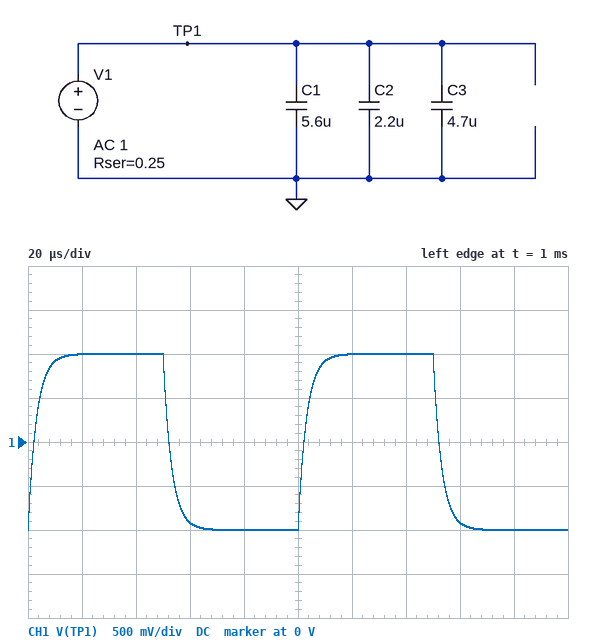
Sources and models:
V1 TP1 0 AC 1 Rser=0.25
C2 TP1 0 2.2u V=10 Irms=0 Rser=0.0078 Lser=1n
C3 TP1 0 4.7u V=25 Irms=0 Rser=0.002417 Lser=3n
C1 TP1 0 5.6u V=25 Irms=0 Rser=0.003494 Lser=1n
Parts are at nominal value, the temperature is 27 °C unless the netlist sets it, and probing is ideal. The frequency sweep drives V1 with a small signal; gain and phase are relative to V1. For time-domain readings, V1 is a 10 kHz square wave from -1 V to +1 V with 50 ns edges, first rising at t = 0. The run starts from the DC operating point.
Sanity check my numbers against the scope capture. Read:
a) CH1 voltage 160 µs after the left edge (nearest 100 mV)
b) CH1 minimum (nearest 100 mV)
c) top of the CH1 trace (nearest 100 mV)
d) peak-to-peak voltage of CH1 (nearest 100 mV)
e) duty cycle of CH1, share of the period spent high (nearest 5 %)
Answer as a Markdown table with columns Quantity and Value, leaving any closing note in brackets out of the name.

| Quantity | Value |
|---|---|
| CH1 voltage 160 µs after the left edge | -900 mV |
| CH1 minimum | -1.0 V |
| top of the CH1 trace | 1.0 V |
| peak-to-peak voltage of CH1 | 2.0 V |
| duty cycle of CH1, share of the period spent high | 50 % |
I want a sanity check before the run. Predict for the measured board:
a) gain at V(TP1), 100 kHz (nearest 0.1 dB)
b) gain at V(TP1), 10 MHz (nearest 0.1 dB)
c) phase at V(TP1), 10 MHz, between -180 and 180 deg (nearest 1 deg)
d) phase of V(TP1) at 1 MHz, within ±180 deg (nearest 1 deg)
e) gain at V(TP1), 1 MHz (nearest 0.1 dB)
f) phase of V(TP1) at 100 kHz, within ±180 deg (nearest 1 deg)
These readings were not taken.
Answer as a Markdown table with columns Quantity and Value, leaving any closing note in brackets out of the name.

| Quantity | Value |
|---|---|
| gain at V(TP1), 100 kHz | -6.9 dB |
| gain at V(TP1), 10 MHz | -20.1 dB |
| phase at V(TP1), 10 MHz, between -180 and 180 deg | 79 deg |
| phase of V(TP1) at 1 MHz, within ±180 deg | -79 deg |
| gain at V(TP1), 1 MHz | -30.0 dB |
| phase of V(TP1) at 100 kHz, within ±180 deg | -63 deg |
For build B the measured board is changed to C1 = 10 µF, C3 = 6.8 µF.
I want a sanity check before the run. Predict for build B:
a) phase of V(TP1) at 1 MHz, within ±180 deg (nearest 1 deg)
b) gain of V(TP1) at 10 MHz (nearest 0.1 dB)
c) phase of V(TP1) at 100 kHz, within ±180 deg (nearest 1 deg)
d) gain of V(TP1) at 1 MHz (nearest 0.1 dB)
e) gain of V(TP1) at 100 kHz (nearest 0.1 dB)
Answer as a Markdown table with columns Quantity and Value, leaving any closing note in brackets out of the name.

| Quantity | Value |
|---|---|
| phase of V(TP1) at 1 MHz, within ±180 deg | -65 deg |
| gain of V(TP1) at 10 MHz | -20.0 dB |
| phase of V(TP1) at 100 kHz, within ±180 deg | -71 deg |
| gain of V(TP1) at 1 MHz | -37.7 dB |
| gain of V(TP1) at 100 kHz | -10.0 dB |
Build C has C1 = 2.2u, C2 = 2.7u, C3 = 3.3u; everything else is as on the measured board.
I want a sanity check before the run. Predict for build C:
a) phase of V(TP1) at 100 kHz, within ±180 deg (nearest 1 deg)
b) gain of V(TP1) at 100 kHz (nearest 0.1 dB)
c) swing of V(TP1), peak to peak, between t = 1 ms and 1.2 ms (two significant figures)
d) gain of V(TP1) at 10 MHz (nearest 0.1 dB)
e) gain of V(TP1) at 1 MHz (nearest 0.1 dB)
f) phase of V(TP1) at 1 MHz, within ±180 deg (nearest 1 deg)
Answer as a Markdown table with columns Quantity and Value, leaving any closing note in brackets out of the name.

| Quantity | Value |
|---|---|
| phase of V(TP1) at 100 kHz, within ±180 deg | -52 deg |
| gain of V(TP1) at 100 kHz | -4.3 dB |
| swing of V(TP1), peak to peak, between t = 1 ms and 1.2 ms | 2.0 V |
| gain of V(TP1) at 10 MHz | -20.3 dB |
| gain of V(TP1) at 1 MHz | -24.6 dB |
| phase of V(TP1) at 1 MHz, within ±180 deg | -81 deg |
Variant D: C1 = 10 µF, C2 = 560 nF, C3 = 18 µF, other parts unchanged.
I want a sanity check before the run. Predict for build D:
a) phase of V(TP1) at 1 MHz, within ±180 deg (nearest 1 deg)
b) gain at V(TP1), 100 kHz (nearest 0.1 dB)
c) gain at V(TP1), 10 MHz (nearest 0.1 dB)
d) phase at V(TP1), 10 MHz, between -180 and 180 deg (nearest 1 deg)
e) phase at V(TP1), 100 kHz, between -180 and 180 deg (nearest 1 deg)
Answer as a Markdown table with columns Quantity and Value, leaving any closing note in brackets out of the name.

| Quantity | Value |
|---|---|
| phase of V(TP1) at 1 MHz, within ±180 deg | -1 deg |
| gain at V(TP1), 100 kHz | -13.4 dB |
| gain at V(TP1), 10 MHz | -22.0 dB |
| phase at V(TP1), 10 MHz, between -180 and 180 deg | 77 deg |
| phase at V(TP1), 100 kHz, between -180 and 180 deg | -76 deg |
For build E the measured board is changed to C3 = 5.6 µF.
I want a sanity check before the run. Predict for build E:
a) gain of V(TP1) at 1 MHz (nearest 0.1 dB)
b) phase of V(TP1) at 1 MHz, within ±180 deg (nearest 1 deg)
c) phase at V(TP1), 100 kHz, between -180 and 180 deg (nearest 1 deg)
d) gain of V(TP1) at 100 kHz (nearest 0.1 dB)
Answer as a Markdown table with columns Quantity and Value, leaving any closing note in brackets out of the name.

| Quantity | Value |
|---|---|
| gain of V(TP1) at 1 MHz | -32.1 dB |
| phase of V(TP1) at 1 MHz, within ±180 deg | -77 deg |
| phase at V(TP1), 100 kHz, between -180 and 180 deg | -64 deg |
| gain of V(TP1) at 100 kHz | -7.4 dB |
